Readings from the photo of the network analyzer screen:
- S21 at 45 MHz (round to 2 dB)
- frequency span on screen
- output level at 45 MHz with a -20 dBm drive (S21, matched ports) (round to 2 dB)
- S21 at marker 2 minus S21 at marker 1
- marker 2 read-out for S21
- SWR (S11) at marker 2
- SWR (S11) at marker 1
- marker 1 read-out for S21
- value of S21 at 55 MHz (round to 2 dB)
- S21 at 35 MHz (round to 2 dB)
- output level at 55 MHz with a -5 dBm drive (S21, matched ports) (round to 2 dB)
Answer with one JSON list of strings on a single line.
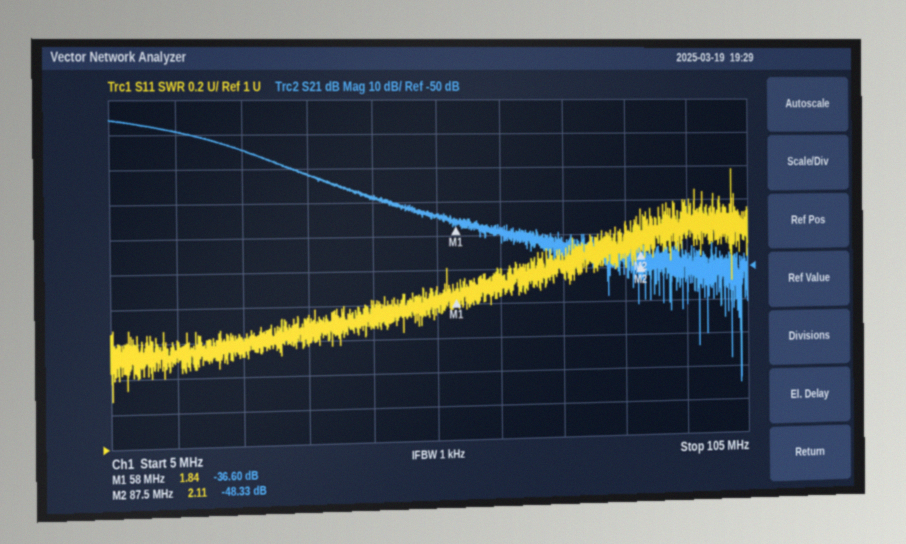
["-28 dB", "100 MHz", "-48 dBm", "-11.73 dB", "-48.33 dB", "2.11", "1.84", "-36.60 dB", "-34 dB", "-22 dB", "-38 dBm"]
